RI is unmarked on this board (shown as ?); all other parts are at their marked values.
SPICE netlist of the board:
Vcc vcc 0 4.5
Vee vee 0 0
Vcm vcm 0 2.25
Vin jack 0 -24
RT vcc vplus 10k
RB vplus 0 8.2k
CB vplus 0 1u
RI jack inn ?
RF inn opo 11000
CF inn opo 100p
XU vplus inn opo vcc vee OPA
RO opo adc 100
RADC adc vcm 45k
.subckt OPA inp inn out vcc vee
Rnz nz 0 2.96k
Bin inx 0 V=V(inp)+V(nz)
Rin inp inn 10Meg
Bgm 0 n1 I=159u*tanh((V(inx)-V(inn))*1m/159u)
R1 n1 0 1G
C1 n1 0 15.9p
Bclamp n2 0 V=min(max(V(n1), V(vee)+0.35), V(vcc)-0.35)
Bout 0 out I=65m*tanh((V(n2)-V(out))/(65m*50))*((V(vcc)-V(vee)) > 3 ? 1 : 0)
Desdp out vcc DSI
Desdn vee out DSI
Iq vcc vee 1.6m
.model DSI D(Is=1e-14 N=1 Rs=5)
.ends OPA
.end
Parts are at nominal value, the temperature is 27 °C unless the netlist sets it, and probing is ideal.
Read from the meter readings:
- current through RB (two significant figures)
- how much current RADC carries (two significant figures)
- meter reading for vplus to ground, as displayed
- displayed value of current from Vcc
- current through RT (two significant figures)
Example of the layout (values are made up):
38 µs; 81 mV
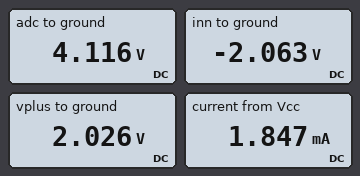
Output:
250 µA; 41 µA; 2.026 V; 1.847 mA; 250 µA
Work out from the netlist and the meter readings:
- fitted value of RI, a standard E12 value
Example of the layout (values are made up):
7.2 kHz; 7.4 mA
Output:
39 kΩ
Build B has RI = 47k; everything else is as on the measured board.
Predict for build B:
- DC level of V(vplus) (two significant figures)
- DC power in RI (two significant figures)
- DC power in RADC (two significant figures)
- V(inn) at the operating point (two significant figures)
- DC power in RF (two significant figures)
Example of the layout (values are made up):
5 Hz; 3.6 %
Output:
2.0 V; 11 mW; 78 µW; -1.2 V; 2.6 mW
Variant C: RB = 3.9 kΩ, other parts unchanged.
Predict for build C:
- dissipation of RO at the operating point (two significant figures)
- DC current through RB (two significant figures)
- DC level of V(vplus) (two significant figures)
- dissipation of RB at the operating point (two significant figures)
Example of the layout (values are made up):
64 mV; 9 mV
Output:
170 nW; 320 µA; 1.3 V; 410 µW
